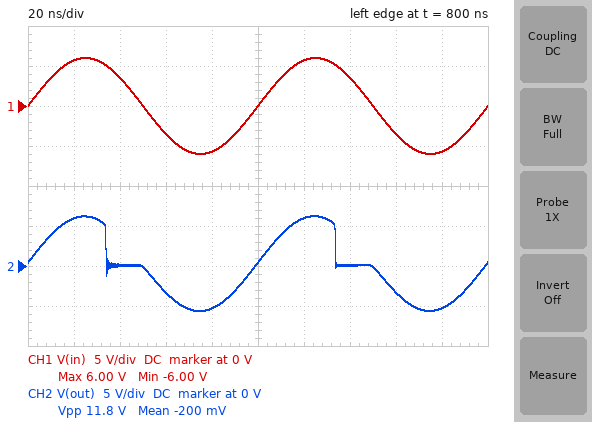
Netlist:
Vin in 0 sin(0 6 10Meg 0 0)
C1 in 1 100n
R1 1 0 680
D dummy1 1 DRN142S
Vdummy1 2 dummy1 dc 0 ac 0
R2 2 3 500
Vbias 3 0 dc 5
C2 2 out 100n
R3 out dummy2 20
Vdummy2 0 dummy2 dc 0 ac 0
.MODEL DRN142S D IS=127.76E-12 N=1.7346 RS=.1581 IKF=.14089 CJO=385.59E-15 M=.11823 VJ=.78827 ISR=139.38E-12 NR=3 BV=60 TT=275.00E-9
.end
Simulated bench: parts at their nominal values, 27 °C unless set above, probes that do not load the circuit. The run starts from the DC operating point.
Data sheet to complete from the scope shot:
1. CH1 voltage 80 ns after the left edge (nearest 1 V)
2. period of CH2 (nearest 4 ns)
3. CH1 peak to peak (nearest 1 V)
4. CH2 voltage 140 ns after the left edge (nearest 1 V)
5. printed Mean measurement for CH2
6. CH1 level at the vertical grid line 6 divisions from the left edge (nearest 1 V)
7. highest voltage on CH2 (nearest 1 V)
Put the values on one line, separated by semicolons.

-6 V; 100 ns; 12 V; 0 V; -200 mV; 6 V; 6 V
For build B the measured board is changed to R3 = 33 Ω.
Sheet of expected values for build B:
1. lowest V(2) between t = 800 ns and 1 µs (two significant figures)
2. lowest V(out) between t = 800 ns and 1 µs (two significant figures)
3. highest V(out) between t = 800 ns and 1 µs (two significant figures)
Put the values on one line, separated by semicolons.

-2.6 V; -5.8 V; 6.1 V
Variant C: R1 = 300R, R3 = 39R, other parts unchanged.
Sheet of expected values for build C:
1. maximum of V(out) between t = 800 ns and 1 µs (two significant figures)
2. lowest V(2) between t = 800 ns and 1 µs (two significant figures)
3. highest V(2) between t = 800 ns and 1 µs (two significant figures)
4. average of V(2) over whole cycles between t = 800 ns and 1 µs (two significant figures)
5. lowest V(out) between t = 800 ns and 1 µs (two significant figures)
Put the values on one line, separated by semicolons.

6.1 V; -3.5 V; 8.4 V; 2.2 V; -5.9 V
